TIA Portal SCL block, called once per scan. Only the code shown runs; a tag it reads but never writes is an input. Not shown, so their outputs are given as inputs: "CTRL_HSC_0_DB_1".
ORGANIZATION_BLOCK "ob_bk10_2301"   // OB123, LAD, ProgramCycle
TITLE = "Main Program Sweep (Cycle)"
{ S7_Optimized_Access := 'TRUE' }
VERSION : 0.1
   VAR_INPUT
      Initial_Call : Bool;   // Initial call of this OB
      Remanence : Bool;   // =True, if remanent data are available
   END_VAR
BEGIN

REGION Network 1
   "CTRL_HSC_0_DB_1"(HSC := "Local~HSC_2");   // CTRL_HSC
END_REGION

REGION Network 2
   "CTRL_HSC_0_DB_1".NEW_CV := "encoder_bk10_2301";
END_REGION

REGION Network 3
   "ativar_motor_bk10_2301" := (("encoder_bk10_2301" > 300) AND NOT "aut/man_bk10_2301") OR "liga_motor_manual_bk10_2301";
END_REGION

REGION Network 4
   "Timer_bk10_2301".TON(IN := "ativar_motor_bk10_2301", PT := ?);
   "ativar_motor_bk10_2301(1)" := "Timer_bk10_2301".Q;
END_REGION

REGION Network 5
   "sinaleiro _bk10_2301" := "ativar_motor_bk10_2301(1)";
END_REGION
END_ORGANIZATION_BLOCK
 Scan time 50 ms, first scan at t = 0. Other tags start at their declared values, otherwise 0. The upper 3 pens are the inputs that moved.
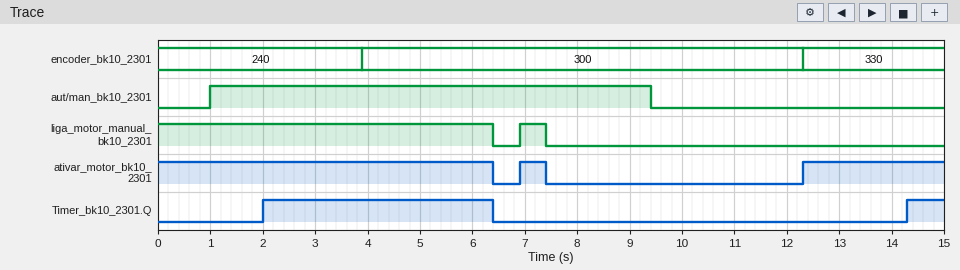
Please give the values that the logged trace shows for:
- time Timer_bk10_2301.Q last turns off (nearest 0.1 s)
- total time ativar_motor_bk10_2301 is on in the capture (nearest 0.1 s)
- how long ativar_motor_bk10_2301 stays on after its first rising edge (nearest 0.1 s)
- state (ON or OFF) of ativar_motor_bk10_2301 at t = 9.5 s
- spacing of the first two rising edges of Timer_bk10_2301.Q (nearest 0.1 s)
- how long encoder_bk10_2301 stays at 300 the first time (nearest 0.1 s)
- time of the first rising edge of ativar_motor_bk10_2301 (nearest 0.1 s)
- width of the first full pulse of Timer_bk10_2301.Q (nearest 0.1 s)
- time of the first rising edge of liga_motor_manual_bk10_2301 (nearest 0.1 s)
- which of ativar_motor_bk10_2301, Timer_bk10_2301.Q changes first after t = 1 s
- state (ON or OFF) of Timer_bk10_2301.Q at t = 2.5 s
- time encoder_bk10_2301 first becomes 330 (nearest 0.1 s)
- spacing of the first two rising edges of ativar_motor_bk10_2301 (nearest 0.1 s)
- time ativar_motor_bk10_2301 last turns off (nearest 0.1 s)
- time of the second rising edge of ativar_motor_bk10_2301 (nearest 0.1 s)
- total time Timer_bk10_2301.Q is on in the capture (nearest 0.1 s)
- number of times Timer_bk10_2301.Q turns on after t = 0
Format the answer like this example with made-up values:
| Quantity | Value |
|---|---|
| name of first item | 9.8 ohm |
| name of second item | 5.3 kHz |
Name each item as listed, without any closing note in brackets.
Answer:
| Quantity | Value |
|---|---|
| time Timer_bk10_2301.Q last turns off | 6.4 s |
| total time ativar_motor_bk10_2301 is on in the capture | 9.6 s |
| how long ativar_motor_bk10_2301 stays on after its first rising edge | 0.5 s |
| state (ON or OFF) of ativar_motor_bk10_2301 at t = 9.5 s | OFF |
| spacing of the first two rising edges of Timer_bk10_2301.Q | 12.3 s |
| how long encoder_bk10_2301 stays at 300 the first time | 8.4 s |
| time of the first rising edge of ativar_motor_bk10_2301 | 6.9 s |
| width of the first full pulse of Timer_bk10_2301.Q | 4.4 s |
| time of the first rising edge of liga_motor_manual_bk10_2301 | 6.9 s |
| which of ativar_motor_bk10_2301, Timer_bk10_2301.Q changes first after t = 1 s | Timer_bk10_2301.Q |
| state (ON or OFF) of Timer_bk10_2301.Q at t = 2.5 s | ON |
| time encoder_bk10_2301 first becomes 330 | 12.3 s |
| spacing of the first two rising edges of ativar_motor_bk10_2301 | 5.4 s |
| time ativar_motor_bk10_2301 last turns off | 7.4 s |
| time of the second rising edge of ativar_motor_bk10_2301 | 12.3 s |
| total time Timer_bk10_2301.Q is on in the capture | 5.1 s |
| number of times Timer_bk10_2301.Q turns on after t = 0 | 2 |
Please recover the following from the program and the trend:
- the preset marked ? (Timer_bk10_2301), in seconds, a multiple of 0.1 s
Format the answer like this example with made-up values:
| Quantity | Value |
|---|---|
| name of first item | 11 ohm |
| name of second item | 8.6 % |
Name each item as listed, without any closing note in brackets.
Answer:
| Quantity | Value |
|---|---|
| the preset marked ? (Timer_bk10_2301), in seconds, a multiple of 0.1 s | 2.0 s |
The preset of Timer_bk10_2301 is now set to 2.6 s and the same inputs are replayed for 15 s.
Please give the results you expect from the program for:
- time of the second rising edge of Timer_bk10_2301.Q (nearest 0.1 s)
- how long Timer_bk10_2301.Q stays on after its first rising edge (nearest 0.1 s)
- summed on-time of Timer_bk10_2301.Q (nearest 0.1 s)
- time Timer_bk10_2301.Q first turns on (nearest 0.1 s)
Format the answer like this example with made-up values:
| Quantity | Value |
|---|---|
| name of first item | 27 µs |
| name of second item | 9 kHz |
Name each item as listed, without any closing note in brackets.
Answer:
| Quantity | Value |
|---|---|
| time of the second rising edge of Timer_bk10_2301.Q | 14.9 s |
| how long Timer_bk10_2301.Q stays on after its first rising edge | 3.8 s |
| summed on-time of Timer_bk10_2301.Q | 3.9 s |
| time Timer_bk10_2301.Q first turns on | 2.6 s |
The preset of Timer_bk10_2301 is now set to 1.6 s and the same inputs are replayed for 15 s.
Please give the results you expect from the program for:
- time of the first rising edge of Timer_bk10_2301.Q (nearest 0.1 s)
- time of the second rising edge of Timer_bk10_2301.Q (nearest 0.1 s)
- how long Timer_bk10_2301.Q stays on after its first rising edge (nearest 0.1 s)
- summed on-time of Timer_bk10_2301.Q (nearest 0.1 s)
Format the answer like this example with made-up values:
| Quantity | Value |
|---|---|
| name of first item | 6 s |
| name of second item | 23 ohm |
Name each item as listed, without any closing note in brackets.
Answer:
| Quantity | Value |
|---|---|
| time of the first rising edge of Timer_bk10_2301.Q | 1.6 s |
| time of the second rising edge of Timer_bk10_2301.Q | 13.9 s |
| how long Timer_bk10_2301.Q stays on after its first rising edge | 4.8 s |
| summed on-time of Timer_bk10_2301.Q | 5.9 s |
